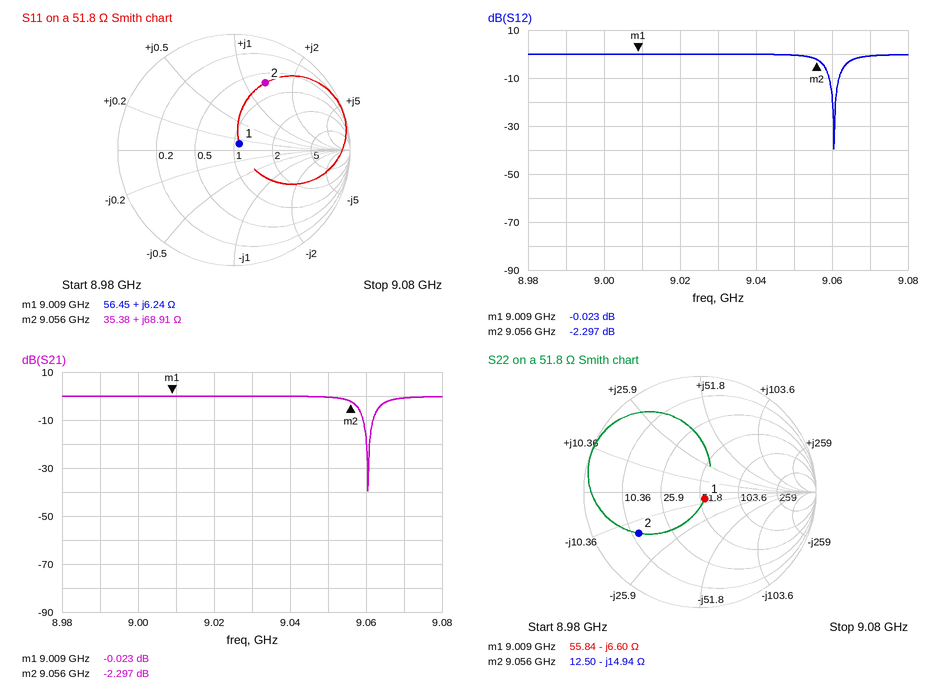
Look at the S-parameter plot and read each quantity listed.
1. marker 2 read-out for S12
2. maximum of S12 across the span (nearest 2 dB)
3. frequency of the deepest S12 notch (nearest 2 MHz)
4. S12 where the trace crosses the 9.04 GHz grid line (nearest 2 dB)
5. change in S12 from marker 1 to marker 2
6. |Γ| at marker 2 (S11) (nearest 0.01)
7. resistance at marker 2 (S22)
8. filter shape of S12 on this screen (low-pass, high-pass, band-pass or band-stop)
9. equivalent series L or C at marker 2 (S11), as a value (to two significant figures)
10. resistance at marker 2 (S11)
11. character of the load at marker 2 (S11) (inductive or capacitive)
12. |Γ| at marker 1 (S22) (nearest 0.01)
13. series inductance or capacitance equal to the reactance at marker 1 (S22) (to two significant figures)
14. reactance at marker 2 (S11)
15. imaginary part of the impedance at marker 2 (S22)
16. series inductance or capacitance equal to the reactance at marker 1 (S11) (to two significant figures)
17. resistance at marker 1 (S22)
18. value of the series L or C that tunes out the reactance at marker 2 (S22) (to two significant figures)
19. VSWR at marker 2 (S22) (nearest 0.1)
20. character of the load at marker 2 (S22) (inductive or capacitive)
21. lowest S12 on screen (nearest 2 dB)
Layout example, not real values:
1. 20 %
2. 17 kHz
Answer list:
1. -2.297 dB
2. 0 dB
3. 9.060 GHz
4. 0 dB
5. -2.274 dB
6. 0.64
7. 12.50 Ω
8. band-stop
9. 1.2 nH
10. 35.38 Ω
11. inductive
12. 0.07
13. 2.7 pF
14. +68.91 Ω
15. -14.94 Ω
16. 110 pH
17. 55.84 Ω
18. 260 pH
19. 4.5
20. capacitive
21. -40 dB
